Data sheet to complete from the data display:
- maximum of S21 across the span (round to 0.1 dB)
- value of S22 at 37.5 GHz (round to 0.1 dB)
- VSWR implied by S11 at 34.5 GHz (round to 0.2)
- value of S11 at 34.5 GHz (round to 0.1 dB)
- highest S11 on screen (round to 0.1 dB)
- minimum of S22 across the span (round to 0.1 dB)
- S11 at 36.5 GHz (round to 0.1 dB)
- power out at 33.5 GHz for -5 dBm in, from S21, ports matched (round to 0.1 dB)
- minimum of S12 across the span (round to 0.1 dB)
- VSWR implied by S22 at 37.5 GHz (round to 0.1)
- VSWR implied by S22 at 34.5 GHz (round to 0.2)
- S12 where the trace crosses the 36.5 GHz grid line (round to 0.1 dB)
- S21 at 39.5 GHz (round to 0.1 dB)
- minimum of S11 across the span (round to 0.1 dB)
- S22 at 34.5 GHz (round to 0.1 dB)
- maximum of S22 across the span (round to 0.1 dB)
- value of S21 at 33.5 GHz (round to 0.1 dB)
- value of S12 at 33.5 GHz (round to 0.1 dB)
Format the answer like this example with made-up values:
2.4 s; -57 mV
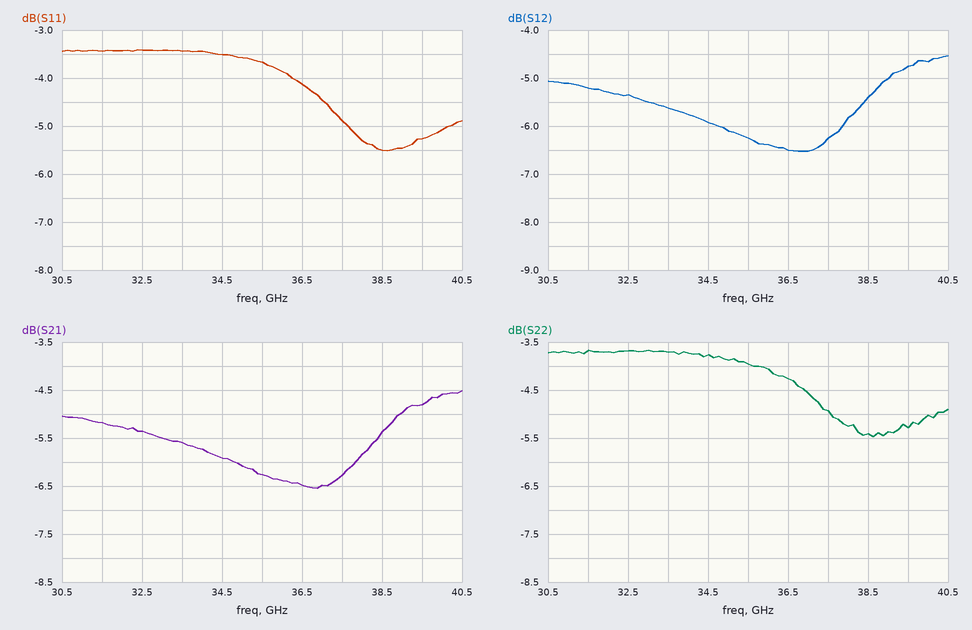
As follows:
-4.5 dB; -4.9 dB; 5.0; -3.5 dB; -3.4 dB; -5.5 dB; -4.1 dB; -10.6 dBm; -6.5 dB; 3.6; 4.6; -6.5 dB; -4.8 dB; -5.5 dB; -3.8 dB; -3.7 dB; -5.6 dB; -5.6 dB
